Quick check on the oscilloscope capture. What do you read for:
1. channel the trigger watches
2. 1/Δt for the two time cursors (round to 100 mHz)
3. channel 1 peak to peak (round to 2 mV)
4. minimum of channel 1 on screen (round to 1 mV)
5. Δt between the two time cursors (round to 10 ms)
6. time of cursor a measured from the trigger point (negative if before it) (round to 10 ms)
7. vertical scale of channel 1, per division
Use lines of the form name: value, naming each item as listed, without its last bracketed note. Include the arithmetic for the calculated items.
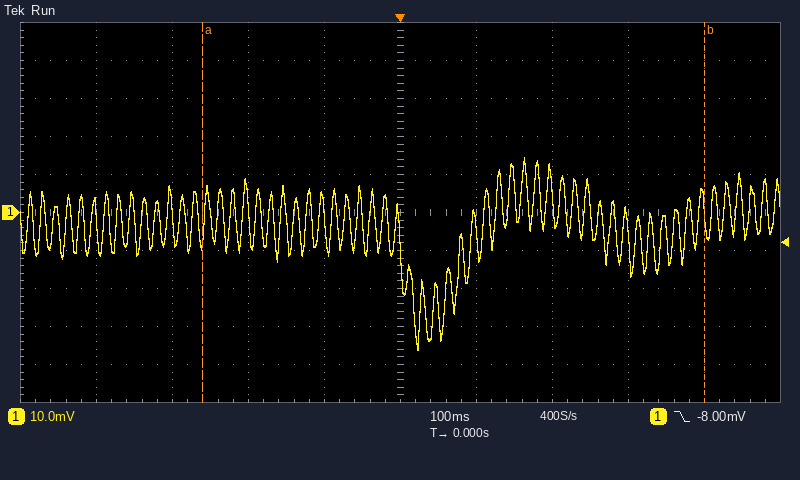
channel the trigger watches: channel 1
1/Δt for the two time cursors: 1 / 660 ms ≈ 1.5 Hz
channel 1 peak to peak: 50 mV
minimum of channel 1 on screen: -36 mV
Δt between the two time cursors: 660 ms
time of cursor a measured from the trigger point (negative if before it): -260 ms
vertical scale of channel 1, per division: 10 mV
